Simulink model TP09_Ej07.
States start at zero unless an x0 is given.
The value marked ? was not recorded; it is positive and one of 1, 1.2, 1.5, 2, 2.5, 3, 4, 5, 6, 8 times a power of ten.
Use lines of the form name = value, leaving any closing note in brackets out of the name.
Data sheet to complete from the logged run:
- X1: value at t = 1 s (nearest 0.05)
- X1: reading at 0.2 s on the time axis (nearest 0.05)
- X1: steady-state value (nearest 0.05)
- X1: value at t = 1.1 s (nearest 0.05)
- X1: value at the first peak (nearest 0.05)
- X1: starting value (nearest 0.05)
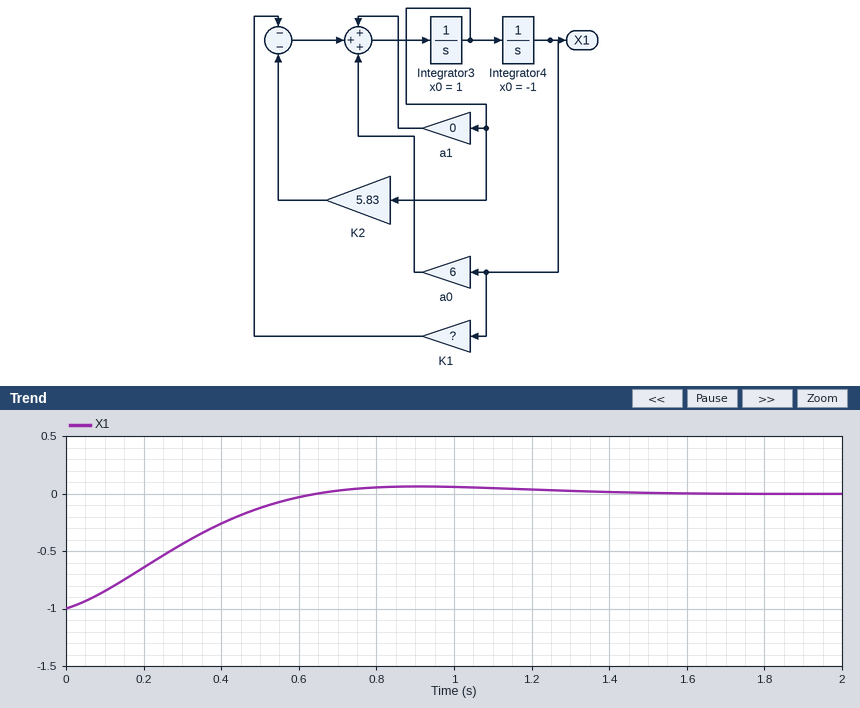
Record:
X1: value at t = 1 s = 0.05
X1: reading at 0.2 s on the time axis = -0.65
X1: steady-state value = 0.00
X1: value at t = 1.1 s = 0.05
X1: value at the first peak = 0.05
X1: starting value = -1.00
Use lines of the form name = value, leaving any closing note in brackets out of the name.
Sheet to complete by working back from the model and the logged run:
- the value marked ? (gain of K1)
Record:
the value marked ? = 25
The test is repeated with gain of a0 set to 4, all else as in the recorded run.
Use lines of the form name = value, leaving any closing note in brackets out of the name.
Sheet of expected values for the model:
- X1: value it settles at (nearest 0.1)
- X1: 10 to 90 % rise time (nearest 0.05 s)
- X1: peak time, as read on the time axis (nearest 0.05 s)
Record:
X1: value it settles at = 0.0
X1: 10 to 90 % rise time = 0.40 s
X1: peak time, as read on the time axis = 0.85 s
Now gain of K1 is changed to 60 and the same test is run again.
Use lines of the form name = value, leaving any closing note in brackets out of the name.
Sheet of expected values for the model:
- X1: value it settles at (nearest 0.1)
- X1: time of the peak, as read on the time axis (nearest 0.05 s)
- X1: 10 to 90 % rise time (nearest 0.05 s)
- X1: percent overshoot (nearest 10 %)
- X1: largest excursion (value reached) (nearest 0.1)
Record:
X1: value it settles at = 0.0
X1: time of the peak, as read on the time axis = 0.45 s
X1: 10 to 90 % rise time = 0.20 s
X1: percent overshoot = 30 %
X1: largest excursion (value reached) = 0.3
